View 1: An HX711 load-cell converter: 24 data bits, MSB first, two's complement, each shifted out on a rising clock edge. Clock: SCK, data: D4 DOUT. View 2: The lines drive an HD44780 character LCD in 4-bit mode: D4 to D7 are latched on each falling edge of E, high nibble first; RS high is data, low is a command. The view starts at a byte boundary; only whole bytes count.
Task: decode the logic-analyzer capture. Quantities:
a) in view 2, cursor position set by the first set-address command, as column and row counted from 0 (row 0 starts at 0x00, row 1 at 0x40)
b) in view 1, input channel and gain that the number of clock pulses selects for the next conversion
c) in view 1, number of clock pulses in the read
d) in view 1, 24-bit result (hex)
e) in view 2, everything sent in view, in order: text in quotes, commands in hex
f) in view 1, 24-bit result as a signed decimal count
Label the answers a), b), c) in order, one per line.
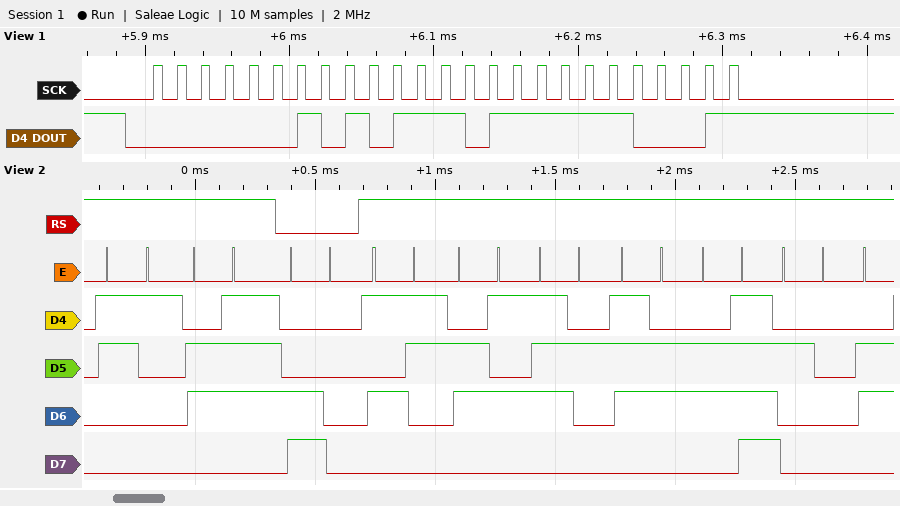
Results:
a) column 0, row 1
b) channel A, gain 128
c) 25
d) 0x02BBF1
e) "1g" 0xC0 "Servo "
f) 179185
